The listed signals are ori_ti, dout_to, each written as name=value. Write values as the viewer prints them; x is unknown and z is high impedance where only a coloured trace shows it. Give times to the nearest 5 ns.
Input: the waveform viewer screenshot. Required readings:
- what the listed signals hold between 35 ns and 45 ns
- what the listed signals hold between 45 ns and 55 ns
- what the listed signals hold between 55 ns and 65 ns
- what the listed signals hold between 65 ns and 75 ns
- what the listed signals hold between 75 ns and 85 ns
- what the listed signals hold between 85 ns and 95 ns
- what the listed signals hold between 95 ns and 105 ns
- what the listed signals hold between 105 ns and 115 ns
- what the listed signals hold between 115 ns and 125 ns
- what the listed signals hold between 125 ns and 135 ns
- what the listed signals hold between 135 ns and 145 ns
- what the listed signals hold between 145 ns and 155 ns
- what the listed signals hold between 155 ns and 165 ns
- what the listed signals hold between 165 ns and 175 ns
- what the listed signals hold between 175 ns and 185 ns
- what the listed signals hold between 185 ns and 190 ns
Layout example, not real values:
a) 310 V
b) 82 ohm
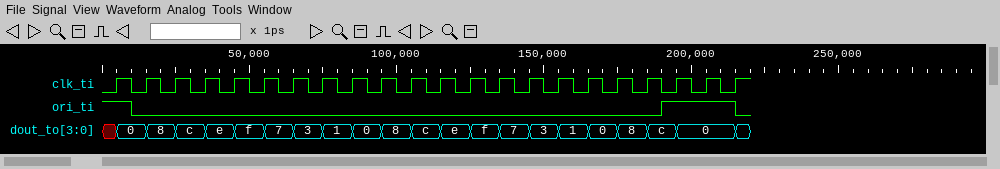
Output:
a) ori_ti=0, dout_to=e
b) ori_ti=0, dout_to=f
c) ori_ti=0, dout_to=7
d) ori_ti=0, dout_to=3
e) ori_ti=0, dout_to=1
f) ori_ti=0, dout_to=0
g) ori_ti=0, dout_to=8
h) ori_ti=0, dout_to=c
i) ori_ti=0, dout_to=e
j) ori_ti=0, dout_to=f
k) ori_ti=0, dout_to=7
l) ori_ti=0, dout_to=3
m) ori_ti=0, dout_to=1
n) ori_ti=0, dout_to=0
o) ori_ti=0, dout_to=8
p) ori_ti=0, dout_to=c
